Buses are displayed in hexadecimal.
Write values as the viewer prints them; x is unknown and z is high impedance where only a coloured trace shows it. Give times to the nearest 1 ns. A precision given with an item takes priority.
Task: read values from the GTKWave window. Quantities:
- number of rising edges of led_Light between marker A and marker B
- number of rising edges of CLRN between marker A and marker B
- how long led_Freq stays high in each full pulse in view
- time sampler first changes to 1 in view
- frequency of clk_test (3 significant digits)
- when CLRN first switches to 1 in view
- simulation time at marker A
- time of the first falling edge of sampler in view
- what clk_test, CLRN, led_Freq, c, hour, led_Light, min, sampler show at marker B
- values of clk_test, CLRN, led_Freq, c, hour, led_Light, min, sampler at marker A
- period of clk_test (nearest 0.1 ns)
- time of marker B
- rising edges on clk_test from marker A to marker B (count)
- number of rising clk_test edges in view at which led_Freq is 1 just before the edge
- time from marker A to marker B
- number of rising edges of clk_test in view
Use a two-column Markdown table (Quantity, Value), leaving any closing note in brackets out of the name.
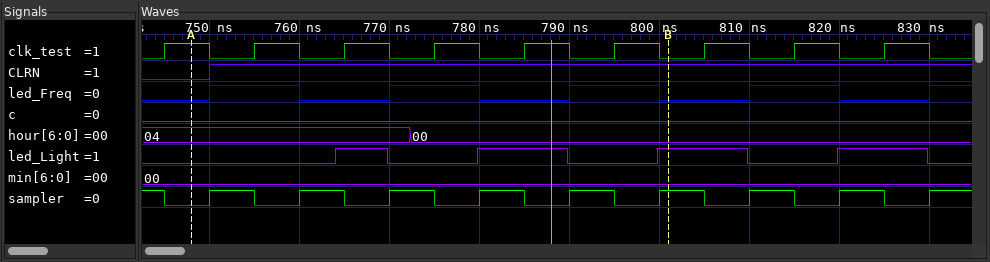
| Quantity | Value |
|---|---|
| number of rising edges of led_Light between marker A and marker B | 3 |
| number of rising edges of CLRN between marker A and marker B | 1 |
| how long led_Freq stays high in each full pulse in view | 10 ns, 10 ns, 10 ns, 10 ns |
| time sampler first changes to 1 in view | 750 ns |
| frequency of clk_test | 100 MHz |
| when CLRN first switches to 1 in view | 750 ns |
| simulation time at marker A | 748 ns |
| time of the first falling edge of sampler in view | 745 ns |
| what clk_test, CLRN, led_Freq, c, hour, led_Light, min, sampler show at marker B | clk_test=0, CLRN=1, led_Freq=0, c=0, hour=00, led_Light=1, min=00, sampler=1 |
| values of clk_test, CLRN, led_Freq, c, hour, led_Light, min, sampler at marker A | clk_test=1, CLRN=0, led_Freq=0, c=0, hour=04, led_Light=0, min=00, sampler=0 |
| period of clk_test | 10 ns |
| time of marker B | 801 ns |
| rising edges on clk_test from marker A to marker B | 5 |
| number of rising clk_test edges in view at which led_Freq is 1 just before the edge | 4 |
| time from marker A to marker B | 53 ns |
| number of rising edges of clk_test in view | 9 |
